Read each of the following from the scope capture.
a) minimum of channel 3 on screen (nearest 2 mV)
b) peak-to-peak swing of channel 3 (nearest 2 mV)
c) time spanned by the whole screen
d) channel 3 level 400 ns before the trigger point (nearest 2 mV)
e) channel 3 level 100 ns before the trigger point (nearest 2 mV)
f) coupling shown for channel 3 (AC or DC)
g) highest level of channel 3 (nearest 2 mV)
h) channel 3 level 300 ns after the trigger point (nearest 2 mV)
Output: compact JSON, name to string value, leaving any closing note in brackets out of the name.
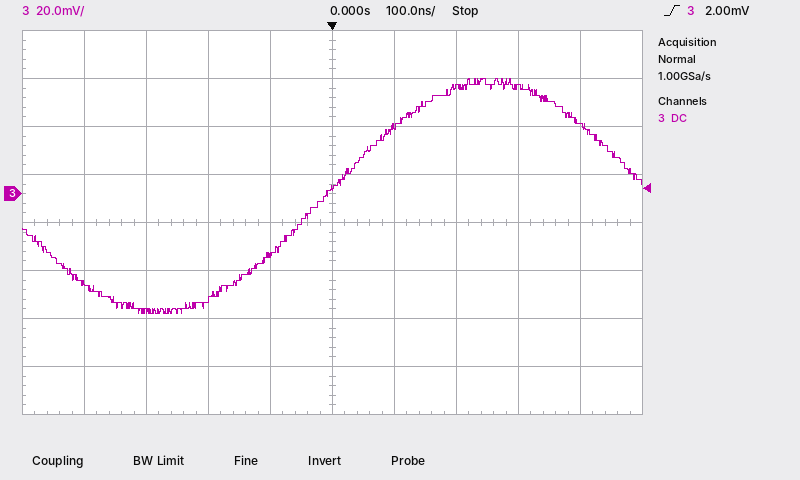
{"minimum of channel 3 on screen": "-50 mV", "peak-to-peak swing of channel 3": "98 mV", "time spanned by the whole screen": "1 µs", "channel 3 level 400 ns before the trigger point": "-38 mV", "channel 3 level 100 ns before the trigger point": "-26 mV", "coupling shown for channel 3": "DC", "highest level of channel 3": "48 mV", "channel 3 level 300 ns after the trigger point": "44 mV"}
